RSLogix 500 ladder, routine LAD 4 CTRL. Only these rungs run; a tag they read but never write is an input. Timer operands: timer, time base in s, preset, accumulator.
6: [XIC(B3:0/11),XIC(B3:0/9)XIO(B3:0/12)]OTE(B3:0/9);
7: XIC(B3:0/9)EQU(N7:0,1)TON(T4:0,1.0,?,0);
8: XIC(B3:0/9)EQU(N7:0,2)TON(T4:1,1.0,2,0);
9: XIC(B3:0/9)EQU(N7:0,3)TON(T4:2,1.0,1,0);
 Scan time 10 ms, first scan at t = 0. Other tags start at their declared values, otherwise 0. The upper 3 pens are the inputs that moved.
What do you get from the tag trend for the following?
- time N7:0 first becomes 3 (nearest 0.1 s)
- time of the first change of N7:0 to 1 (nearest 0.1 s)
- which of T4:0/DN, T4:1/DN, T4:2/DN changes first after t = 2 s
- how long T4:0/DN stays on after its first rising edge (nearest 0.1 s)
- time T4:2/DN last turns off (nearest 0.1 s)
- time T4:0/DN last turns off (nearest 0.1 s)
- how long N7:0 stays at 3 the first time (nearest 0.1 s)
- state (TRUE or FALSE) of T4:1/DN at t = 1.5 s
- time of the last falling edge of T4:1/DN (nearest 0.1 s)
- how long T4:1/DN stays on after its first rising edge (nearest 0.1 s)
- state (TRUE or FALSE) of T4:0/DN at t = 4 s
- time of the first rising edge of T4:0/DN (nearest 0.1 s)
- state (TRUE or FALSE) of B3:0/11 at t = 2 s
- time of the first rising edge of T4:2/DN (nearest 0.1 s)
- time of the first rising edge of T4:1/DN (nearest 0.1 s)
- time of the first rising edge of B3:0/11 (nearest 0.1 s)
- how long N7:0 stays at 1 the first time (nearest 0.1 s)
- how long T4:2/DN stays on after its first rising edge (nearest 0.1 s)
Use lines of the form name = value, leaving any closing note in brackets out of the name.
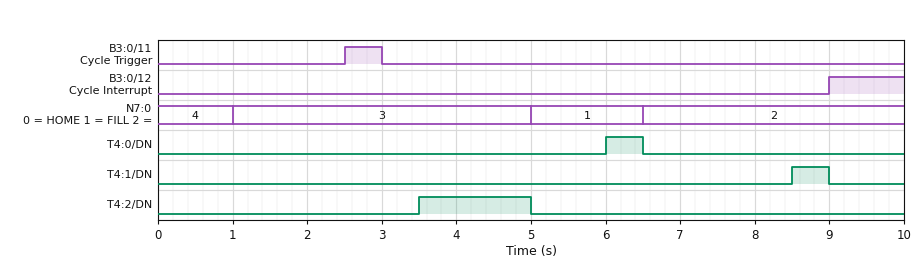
time N7:0 first becomes 3 = 1.0 s
time of the first change of N7:0 to 1 = 5.0 s
which of T4:0/DN, T4:1/DN, T4:2/DN changes first after t = 2 s = T4:2/DN
how long T4:0/DN stays on after its first rising edge = 0.5 s
time T4:2/DN last turns off = 5.0 s
time T4:0/DN last turns off = 6.5 s
how long N7:0 stays at 3 the first time = 4.0 s
state (TRUE or FALSE) of T4:1/DN at t = 1.5 s = FALSE
time of the last falling edge of T4:1/DN = 9.0 s
how long T4:1/DN stays on after its first rising edge = 0.5 s
state (TRUE or FALSE) of T4:0/DN at t = 4 s = FALSE
time of the first rising edge of T4:0/DN = 6.0 s
state (TRUE or FALSE) of B3:0/11 at t = 2 s = FALSE
time of the first rising edge of T4:2/DN = 3.5 s
time of the first rising edge of T4:1/DN = 8.5 s
time of the first rising edge of B3:0/11 = 2.5 s
how long N7:0 stays at 1 the first time = 1.5 s
how long T4:2/DN stays on after its first rising edge = 1.5 s
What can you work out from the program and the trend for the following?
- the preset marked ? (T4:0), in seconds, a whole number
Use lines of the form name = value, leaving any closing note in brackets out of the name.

the preset marked ? (T4:0), in seconds, a whole number = 1 s
